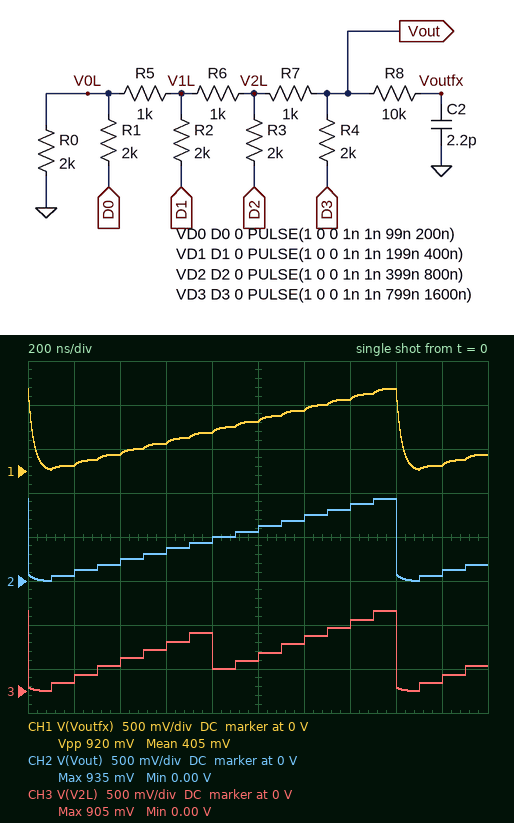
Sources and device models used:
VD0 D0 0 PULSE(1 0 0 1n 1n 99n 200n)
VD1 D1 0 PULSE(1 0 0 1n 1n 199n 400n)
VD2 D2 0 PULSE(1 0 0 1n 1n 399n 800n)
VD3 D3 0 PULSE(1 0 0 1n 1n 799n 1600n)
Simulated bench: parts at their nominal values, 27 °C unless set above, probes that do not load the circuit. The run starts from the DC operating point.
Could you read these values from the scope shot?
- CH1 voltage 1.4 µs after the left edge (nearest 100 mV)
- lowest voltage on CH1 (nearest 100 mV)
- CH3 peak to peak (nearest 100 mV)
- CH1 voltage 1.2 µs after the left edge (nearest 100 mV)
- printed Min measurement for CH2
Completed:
800 mV
0 V
900 mV
700 mV
0.00 V
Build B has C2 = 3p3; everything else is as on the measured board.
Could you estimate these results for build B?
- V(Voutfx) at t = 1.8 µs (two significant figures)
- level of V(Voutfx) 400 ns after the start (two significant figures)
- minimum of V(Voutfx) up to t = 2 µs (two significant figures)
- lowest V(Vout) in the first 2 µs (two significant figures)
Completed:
62 mV
180 mV
59 mV
5.5 mV
